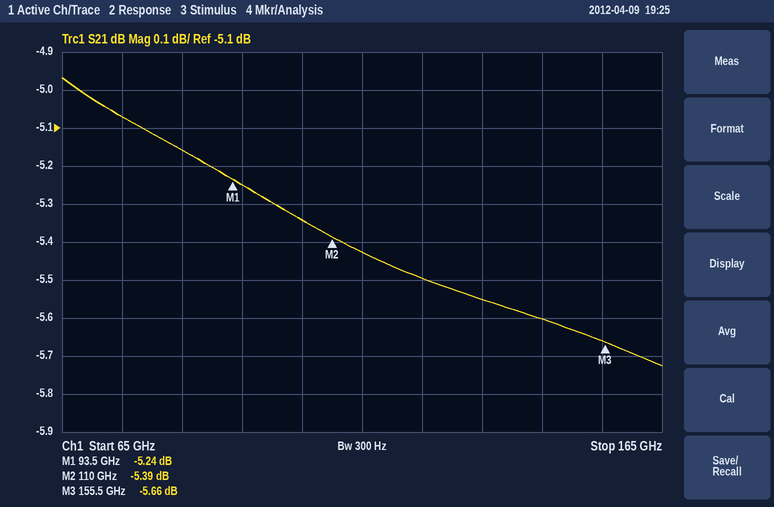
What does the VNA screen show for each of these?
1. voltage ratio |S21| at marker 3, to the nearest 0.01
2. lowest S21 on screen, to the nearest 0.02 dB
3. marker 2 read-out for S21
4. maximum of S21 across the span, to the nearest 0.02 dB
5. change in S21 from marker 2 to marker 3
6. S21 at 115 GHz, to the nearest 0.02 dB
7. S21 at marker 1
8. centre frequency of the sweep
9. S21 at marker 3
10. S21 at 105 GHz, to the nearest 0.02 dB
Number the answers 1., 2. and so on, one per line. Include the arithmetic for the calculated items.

1. 10^(-5.66/20) ≈ 0.52
2. -5.72 dB
3. -5.39 dB
4. -4.96 dB
5. -5.66 − (-5.39) = -0.27 dB
6. -5.42 dB
7. -5.24 dB
8. 115 GHz
9. -5.66 dB
10. -5.34 dB
